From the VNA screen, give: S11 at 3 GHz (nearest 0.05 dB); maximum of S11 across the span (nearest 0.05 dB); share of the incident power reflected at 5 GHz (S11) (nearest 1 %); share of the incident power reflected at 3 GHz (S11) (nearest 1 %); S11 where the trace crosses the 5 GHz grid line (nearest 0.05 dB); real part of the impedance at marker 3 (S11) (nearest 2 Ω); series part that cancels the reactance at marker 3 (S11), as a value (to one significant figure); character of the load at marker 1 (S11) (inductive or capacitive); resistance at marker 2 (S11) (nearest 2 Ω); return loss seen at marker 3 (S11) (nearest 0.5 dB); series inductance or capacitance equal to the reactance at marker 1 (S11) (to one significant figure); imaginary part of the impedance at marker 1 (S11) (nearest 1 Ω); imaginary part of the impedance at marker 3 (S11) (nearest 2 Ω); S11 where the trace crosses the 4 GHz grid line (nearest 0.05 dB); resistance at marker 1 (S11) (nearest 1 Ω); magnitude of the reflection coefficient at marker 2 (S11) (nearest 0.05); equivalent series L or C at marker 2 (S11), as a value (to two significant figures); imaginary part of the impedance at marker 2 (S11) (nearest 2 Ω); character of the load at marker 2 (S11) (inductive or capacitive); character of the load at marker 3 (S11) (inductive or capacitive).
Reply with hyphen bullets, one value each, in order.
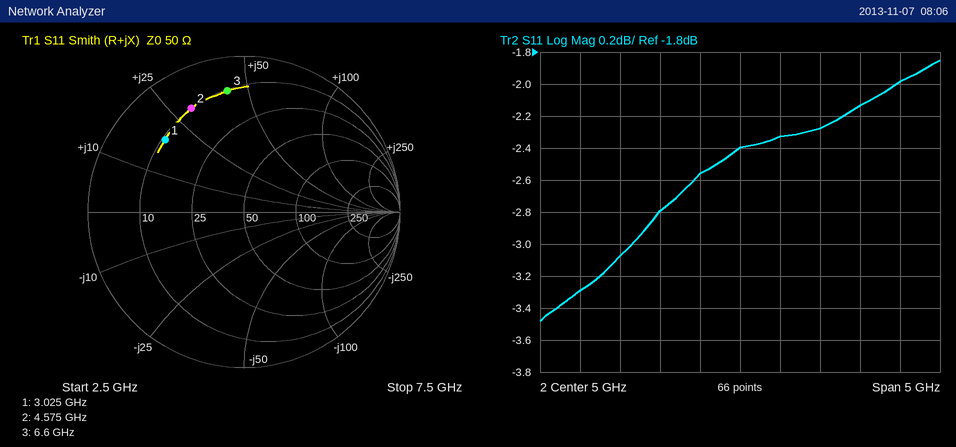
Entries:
- -3.30 dB
- -1.85 dB
- 58 %
- 47 %
- -2.40 dB
- 10 Ω
- 600 fF
- inductive
- 10 Ω
- 2.0 dB
- 1.0 nH
- +19 Ω
- +42 Ω
- -2.80 dB
- 11 Ω
- 0.75
- 1.0 nH
- +30 Ω
- inductive
- inductive
